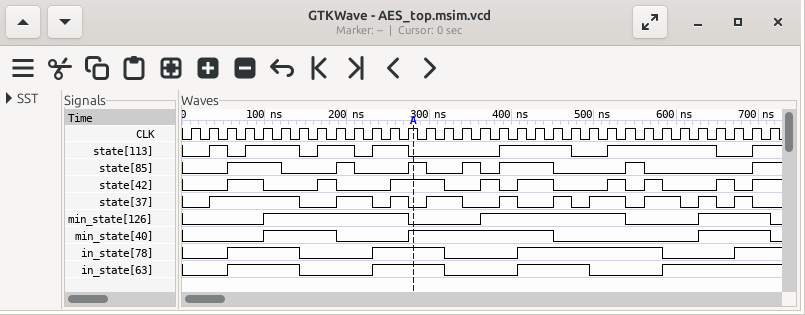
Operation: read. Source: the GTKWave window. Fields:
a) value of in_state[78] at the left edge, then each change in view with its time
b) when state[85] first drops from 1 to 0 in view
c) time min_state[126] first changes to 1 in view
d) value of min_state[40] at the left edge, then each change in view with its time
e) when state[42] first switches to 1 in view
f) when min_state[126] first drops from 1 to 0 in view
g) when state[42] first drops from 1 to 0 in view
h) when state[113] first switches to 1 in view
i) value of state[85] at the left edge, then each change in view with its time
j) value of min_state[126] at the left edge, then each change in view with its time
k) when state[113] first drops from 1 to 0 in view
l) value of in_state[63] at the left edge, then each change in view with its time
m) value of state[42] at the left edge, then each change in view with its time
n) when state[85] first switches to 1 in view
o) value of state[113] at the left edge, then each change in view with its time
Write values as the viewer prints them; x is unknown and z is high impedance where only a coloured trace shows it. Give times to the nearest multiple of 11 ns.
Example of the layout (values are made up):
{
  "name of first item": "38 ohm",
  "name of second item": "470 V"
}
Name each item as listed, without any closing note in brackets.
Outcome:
{
  "value of in_state[78] at the left edge, then each change in view with its time": "0, 1 at 55 ns, 0 at 143 ns, 1 at 231 ns, 0 at 319 ns, 1 at 407 ns, 0 at 583 ns, 1 at 671 ns",
  "when state[85] first drops from 1 to 0 in view": "121 ns",
  "time min_state[126] first changes to 1 in view": "99 ns",
  "value of min_state[40] at the left edge, then each change in view with its time": "0, 1 at 99 ns, 0 at 187 ns, 1 at 275 ns, 0 at 451 ns, 1 at 627 ns, 0 at 715 ns",
  "when state[42] first switches to 1 in view": "55 ns",
  "when min_state[126] first drops from 1 to 0 in view": "275 ns",
  "when state[42] first drops from 1 to 0 in view": "99 ns",
  "when state[113] first switches to 1 in view": "33 ns",
  "value of state[85] at the left edge, then each change in view with its time": "0, 1 at 55 ns, 0 at 121 ns, 1 at 187 ns, 0 at 209 ns, 1 at 275 ns, 0 at 297 ns, 1 at 341 ns, 0 at 363 ns, 1 at 385 ns, 0 at 451 ns, 1 at 539 ns, 0 at 561 ns, 1 at 693 ns",
  "value of min_state[126] at the left edge, then each change in view with its time": "0, 1 at 99 ns, 0 at 275 ns, 1 at 363 ns, 0 at 539 ns, 1 at 627 ns, 0 at 715 ns",
  "when state[113] first drops from 1 to 0 in view": "55 ns",
  "value of in_state[63] at the left edge, then each change in view with its time": "0, 1 at 55 ns, 0 at 143 ns, 1 at 231 ns, 0 at 319 ns, 1 at 407 ns, 0 at 495 ns, 1 at 583 ns",
  "value of state[42] at the left edge, then each change in view with its time": "0, 1 at 55 ns, 0 at 99 ns, 1 at 165 ns, 0 at 187 ns, 1 at 253 ns, 0 at 319 ns, 1 at 363 ns, 0 at 385 ns, 1 at 407 ns, 0 at 451 ns, 1 at 517 ns, 0 at 539 ns, 1 at 561 ns, 0 at 583 ns, 1 at 649 ns, 0 at 671 ns, 1 at 693 ns",
  "when state[85] first switches to 1 in view": "55 ns",
  "value of state[113] at the left edge, then each change in view with its time": "0, 1 at 33 ns, 0 at 55 ns, 1 at 77 ns, 0 at 143 ns, 1 at 165 ns, 0 at 209 ns, 1 at 231 ns, 0 at 275 ns, 1 at 385 ns, 0 at 473 ns, 1 at 517 ns, 0 at 649 ns, 1 at 693 ns"
}
